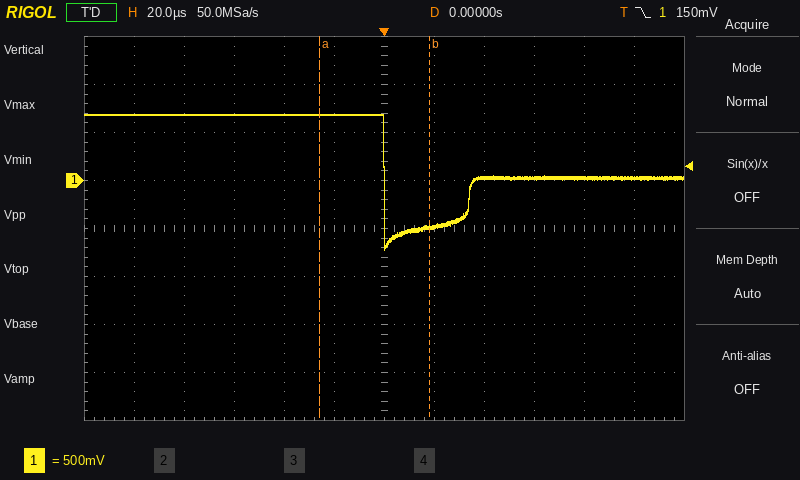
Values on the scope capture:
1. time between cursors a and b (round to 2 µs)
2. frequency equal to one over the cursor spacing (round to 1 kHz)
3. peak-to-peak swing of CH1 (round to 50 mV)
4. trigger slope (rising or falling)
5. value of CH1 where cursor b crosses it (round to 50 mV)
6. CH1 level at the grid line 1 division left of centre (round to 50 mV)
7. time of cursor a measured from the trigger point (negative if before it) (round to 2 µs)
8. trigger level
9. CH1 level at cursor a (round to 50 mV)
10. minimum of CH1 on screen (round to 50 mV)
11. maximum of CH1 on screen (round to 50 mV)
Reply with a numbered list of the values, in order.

1. 44 µs
2. 23 kHz
3. 1.40 V
4. falling
5. -500 mV
6. 700 mV
7. -26 µs
8. 150 mV
9. 700 mV
10. -700 mV
11. 700 mV
